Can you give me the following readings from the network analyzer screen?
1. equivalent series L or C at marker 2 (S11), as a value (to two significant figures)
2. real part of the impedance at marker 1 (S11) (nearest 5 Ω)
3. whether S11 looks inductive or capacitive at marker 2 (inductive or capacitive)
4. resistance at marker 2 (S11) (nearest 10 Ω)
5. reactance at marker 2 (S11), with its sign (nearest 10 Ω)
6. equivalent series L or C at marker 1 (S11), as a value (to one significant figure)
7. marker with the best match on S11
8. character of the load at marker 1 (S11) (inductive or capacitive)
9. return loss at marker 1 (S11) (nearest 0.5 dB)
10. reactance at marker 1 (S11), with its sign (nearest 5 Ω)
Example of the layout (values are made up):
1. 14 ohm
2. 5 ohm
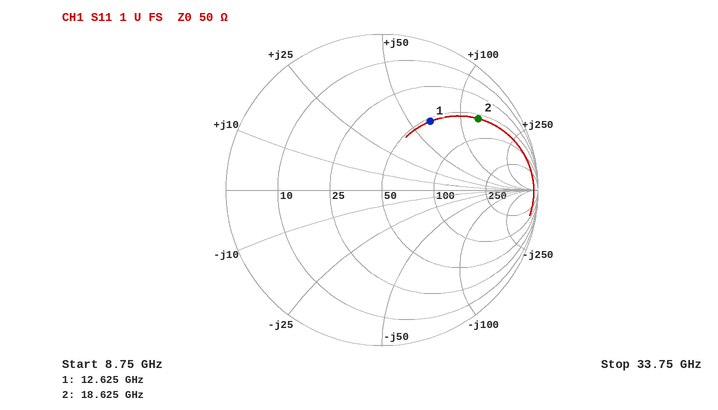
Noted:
1. 1.1 nH
2. 55 Ω
3. inductive
4. 60 Ω
5. +130 Ω
6. 800 pH
7. marker 1
8. inductive
9. 5.5 dB
10. +65 Ω
